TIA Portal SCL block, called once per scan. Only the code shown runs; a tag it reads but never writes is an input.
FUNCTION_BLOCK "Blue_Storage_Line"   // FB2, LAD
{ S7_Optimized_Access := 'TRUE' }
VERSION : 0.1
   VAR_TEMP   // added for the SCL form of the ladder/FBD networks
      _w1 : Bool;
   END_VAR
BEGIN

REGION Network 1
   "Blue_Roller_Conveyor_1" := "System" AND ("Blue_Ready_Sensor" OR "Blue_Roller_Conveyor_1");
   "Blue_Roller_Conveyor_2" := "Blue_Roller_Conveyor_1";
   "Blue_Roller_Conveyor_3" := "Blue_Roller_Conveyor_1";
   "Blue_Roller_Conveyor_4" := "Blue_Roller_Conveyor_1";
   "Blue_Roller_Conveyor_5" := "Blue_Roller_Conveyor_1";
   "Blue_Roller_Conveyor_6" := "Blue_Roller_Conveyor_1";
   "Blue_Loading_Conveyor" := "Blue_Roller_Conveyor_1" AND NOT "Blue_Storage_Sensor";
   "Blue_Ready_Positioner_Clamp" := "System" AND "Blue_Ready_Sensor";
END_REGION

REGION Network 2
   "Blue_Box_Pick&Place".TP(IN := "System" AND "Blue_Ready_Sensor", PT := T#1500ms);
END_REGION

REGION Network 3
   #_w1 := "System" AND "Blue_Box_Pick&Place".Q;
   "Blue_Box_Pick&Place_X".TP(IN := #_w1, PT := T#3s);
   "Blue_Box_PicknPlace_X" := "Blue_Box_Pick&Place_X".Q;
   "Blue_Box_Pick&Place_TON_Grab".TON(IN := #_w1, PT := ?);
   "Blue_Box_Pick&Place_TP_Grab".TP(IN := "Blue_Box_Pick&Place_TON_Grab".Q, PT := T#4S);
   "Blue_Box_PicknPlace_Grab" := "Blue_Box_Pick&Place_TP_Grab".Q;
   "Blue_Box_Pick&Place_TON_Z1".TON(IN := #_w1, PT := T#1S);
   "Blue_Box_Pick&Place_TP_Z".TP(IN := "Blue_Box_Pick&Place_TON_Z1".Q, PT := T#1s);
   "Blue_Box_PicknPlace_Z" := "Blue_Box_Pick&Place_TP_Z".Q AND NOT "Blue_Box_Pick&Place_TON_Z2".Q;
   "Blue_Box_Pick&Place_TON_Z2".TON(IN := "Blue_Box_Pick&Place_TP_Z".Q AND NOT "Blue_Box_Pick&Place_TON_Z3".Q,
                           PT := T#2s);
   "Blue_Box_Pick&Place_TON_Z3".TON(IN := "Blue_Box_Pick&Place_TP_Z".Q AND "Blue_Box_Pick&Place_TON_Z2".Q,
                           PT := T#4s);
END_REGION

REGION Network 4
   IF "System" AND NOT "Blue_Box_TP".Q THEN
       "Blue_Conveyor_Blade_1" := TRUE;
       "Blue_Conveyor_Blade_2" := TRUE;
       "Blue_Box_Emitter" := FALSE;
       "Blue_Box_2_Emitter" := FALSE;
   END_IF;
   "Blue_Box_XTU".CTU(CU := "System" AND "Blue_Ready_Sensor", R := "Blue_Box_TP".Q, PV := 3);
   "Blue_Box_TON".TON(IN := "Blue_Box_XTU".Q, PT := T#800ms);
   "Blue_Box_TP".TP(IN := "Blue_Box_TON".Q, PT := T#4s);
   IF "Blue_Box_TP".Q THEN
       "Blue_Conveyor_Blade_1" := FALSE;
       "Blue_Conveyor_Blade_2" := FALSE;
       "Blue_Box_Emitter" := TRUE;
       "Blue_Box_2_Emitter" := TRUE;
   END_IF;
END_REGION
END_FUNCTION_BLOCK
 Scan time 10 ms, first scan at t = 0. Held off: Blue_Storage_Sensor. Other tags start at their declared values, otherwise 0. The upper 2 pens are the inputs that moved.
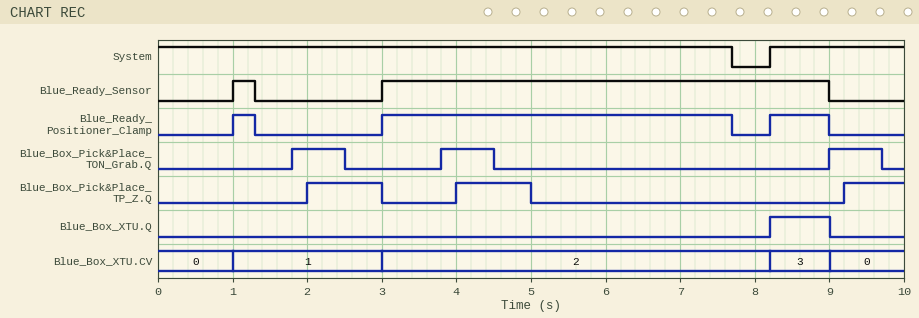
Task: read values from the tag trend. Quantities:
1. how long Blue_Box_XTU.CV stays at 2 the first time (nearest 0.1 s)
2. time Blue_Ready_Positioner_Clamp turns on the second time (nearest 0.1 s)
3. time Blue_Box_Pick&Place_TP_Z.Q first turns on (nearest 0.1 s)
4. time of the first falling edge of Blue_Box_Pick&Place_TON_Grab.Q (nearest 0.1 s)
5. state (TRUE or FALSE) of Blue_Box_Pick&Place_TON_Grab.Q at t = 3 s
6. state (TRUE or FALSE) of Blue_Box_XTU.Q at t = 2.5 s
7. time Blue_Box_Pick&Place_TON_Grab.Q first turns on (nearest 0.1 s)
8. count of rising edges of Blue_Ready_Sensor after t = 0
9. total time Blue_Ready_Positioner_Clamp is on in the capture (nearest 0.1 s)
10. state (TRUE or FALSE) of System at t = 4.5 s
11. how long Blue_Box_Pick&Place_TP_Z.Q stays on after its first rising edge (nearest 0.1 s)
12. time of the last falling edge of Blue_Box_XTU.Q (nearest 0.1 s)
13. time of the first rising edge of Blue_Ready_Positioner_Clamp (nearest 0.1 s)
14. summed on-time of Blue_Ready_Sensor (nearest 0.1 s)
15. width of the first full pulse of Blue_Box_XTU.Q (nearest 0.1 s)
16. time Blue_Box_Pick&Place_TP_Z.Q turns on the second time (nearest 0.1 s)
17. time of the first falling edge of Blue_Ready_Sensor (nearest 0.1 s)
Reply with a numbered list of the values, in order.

1. 5.2 s
2. 3.0 s
3. 2.0 s
4. 2.5 s
5. FALSE
6. FALSE
7. 1.8 s
8. 2
9. 5.8 s
10. TRUE
11. 1.0 s
12. 9.0 s
13. 1.0 s
14. 6.3 s
15. 0.8 s
16. 4.0 s
17. 1.3 s
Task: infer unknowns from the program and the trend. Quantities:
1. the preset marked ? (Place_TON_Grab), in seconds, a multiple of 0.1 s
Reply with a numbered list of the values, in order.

1. 0.8 s
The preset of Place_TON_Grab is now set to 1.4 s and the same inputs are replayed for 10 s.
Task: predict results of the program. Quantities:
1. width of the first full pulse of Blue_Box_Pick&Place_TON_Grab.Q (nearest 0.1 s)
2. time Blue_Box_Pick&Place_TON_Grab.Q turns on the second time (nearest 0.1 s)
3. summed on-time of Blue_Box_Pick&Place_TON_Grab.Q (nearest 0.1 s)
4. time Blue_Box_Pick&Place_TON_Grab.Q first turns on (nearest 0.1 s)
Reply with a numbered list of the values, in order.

1. 0.1 s
2. 4.4 s
3. 0.3 s
4. 2.4 s
